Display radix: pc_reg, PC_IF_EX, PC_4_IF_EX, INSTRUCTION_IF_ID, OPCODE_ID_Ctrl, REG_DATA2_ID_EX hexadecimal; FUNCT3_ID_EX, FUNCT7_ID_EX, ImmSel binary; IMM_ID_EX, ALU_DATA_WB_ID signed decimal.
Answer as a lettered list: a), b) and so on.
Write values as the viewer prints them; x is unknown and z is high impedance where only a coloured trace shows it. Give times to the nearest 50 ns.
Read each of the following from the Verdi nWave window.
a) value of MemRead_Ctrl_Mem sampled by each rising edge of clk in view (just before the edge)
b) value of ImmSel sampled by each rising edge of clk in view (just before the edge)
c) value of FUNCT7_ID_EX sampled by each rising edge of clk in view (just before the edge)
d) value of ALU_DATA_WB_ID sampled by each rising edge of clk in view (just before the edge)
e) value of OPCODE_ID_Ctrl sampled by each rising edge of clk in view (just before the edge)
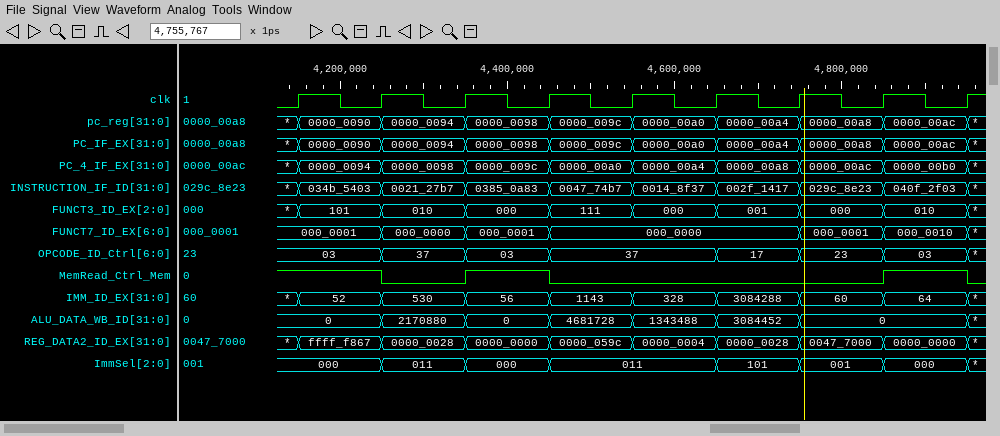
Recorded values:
a) 1 1 0 1 0 0 0 0 1
b) 000, 000, 011, 000, 011, 011, 101, 001, 000
c) 000_0001, 000_0001, 000_0000, 000_0001, 000_0000, 000_0000, 000_0000, 000_0001, 000_0010
d) 0, 0, 2170880, 0, 4681728, 1343488, 3084452, 0, 0
e) 03, 03, 37, 03, 37, 37, 17, 23, 03
